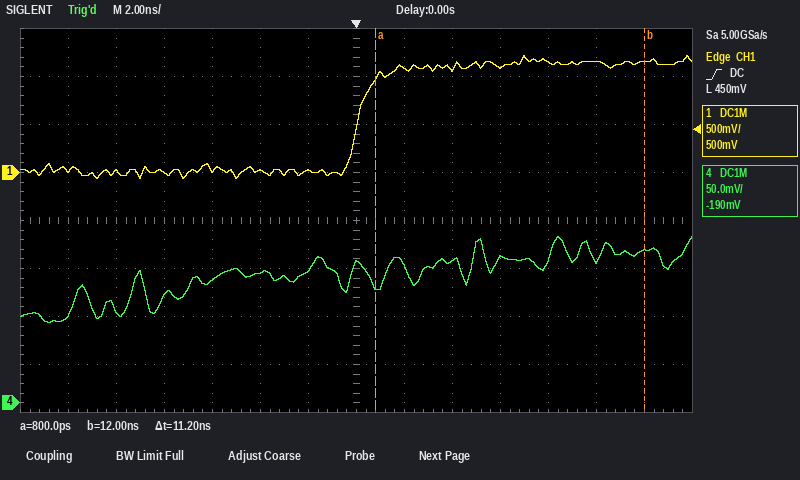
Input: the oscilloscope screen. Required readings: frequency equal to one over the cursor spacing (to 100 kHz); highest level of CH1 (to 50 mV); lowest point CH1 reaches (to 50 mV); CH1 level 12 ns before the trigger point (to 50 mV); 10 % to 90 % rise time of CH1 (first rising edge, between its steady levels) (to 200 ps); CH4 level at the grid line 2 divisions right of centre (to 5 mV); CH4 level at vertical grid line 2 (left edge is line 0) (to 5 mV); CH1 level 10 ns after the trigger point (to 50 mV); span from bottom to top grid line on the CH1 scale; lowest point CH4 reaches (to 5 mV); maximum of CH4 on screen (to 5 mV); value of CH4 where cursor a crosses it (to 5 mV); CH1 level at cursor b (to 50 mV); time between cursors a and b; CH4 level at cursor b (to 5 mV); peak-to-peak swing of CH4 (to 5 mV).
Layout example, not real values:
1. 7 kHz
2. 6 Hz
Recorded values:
1. 89.3 MHz
2. 1.20 V
3. -50 mV
4. 0 mV
5. 1.2 ns
6. 150 mV
7. 95 mV
8. 1.15 V
9. 4 V
10. 85 mV
11. 175 mV
12. 120 mV
13. 1.15 V
14. 11.2 ns
15. 160 mV
16. 90 mV
